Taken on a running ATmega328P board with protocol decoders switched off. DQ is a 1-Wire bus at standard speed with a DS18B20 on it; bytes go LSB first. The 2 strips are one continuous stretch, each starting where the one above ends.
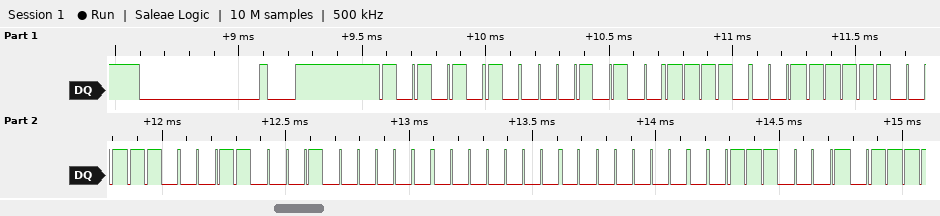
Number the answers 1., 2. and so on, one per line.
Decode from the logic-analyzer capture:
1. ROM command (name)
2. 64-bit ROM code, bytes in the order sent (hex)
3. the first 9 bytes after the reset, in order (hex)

1. Match ROM
2. 28 8F 9F 63 04 00 00 8E
3. 55 28 8F 9F 63 04 00 00 8E
